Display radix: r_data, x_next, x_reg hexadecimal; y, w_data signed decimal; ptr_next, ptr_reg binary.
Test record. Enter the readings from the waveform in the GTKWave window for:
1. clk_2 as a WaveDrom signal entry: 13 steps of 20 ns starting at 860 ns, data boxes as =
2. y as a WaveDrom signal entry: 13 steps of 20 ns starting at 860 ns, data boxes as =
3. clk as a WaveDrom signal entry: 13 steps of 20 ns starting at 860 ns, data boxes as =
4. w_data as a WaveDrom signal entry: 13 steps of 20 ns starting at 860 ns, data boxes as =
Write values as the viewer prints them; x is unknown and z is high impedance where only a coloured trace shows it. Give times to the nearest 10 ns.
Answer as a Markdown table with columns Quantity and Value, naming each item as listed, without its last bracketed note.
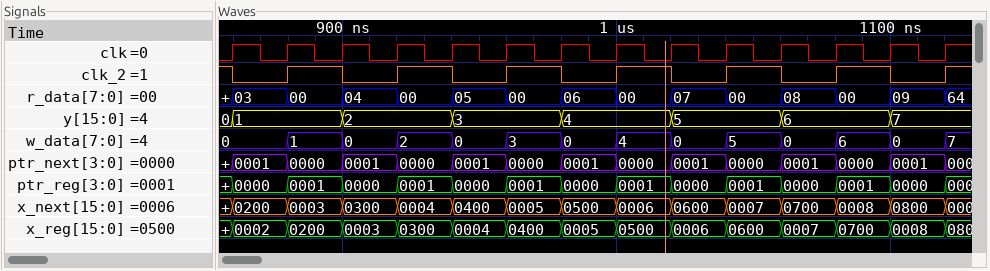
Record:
| Quantity | Value |
|---|---|
| clk_2 as a WaveDrom signal entry: 13 steps of 20 ns starting at 860 ns, data boxes as = | {name: 'clk_2', wave: '0101010101010'} |
| y as a WaveDrom signal entry: 13 steps of 20 ns starting at 860 ns, data boxes as = | {name: 'y', wave: '=.=.=.=.=.=.=', data: '1 2 3 4 5 6 7'} |
| clk as a WaveDrom signal entry: 13 steps of 20 ns starting at 860 ns, data boxes as = | {name: 'clk', wave: 'p............'} |
| w_data as a WaveDrom signal entry: 13 steps of 20 ns starting at 860 ns, data boxes as = | {name: 'w_data', wave: '=============', data: '0 1 0 2 0 3 0 4 0 5 0 6 0'} |
